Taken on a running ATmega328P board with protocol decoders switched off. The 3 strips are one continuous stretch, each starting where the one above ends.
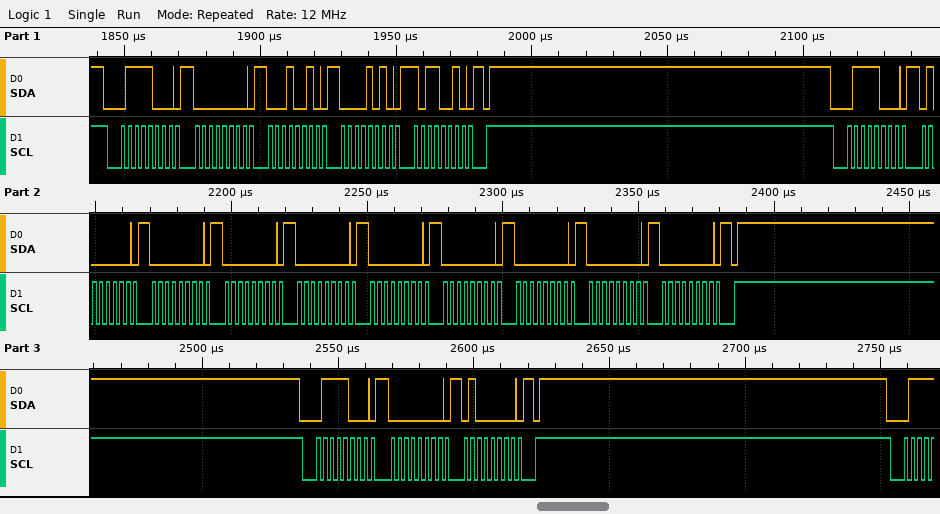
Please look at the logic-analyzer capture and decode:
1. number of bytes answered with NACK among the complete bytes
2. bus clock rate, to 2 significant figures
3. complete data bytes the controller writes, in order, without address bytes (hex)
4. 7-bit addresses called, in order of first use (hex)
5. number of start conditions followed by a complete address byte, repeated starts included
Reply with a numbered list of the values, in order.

1. 0
2. 400 kHz
3. 00 12 0A B2 40 00 00 00 00 00 00 00 00 00 40
4. 0x3C
5. 3
